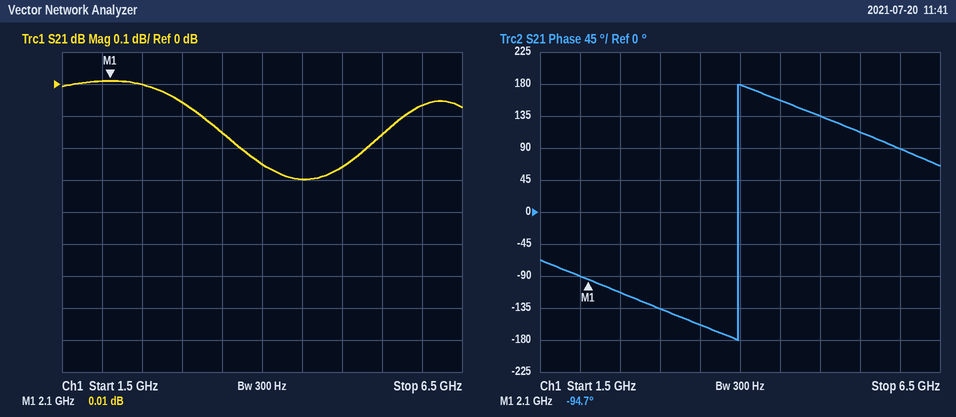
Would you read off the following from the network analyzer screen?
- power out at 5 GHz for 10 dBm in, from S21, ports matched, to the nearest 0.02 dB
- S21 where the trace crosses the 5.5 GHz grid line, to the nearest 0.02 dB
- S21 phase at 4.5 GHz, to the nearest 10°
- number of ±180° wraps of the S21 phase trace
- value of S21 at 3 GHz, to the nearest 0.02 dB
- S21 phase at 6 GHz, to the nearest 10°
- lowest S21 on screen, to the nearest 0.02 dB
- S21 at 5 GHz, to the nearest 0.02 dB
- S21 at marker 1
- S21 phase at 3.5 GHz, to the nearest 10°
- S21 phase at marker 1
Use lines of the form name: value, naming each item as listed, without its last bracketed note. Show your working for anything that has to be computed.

power out at 5 GHz for 10 dBm in, from S21, ports matched, to the nearest 0.02 dB: 10 dBm + (-0.26 dB) = 9.74 dBm
S21 where the trace crosses the 5.5 GHz grid line, to the nearest 0.02 dB: -0.16 dB
S21 phase at 4.5 GHz, to the nearest 10°: 160°
number of ±180° wraps of the S21 phase trace: 1
value of S21 at 3 GHz, to the nearest 0.02 dB: -0.06 dB
S21 phase at 6 GHz, to the nearest 10°: 90°
lowest S21 on screen, to the nearest 0.02 dB: -0.30 dB
S21 at 5 GHz, to the nearest 0.02 dB: -0.26 dB
S21 at marker 1: 0.01 dB
S21 phase at 3.5 GHz, to the nearest 10°: -160°
S21 phase at marker 1: -94.7°
